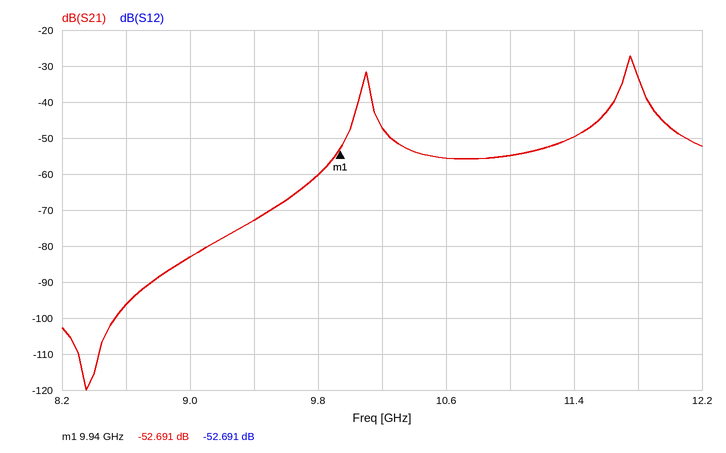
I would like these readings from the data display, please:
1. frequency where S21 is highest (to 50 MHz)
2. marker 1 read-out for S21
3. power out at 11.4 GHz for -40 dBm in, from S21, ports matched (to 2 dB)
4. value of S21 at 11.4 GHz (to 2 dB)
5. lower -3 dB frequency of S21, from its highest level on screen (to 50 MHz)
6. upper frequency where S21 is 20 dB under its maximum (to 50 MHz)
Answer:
11.75 GHz
-52.691 dB
-90 dBm
-50 dB
11.75 GHz
12.00 GHz
